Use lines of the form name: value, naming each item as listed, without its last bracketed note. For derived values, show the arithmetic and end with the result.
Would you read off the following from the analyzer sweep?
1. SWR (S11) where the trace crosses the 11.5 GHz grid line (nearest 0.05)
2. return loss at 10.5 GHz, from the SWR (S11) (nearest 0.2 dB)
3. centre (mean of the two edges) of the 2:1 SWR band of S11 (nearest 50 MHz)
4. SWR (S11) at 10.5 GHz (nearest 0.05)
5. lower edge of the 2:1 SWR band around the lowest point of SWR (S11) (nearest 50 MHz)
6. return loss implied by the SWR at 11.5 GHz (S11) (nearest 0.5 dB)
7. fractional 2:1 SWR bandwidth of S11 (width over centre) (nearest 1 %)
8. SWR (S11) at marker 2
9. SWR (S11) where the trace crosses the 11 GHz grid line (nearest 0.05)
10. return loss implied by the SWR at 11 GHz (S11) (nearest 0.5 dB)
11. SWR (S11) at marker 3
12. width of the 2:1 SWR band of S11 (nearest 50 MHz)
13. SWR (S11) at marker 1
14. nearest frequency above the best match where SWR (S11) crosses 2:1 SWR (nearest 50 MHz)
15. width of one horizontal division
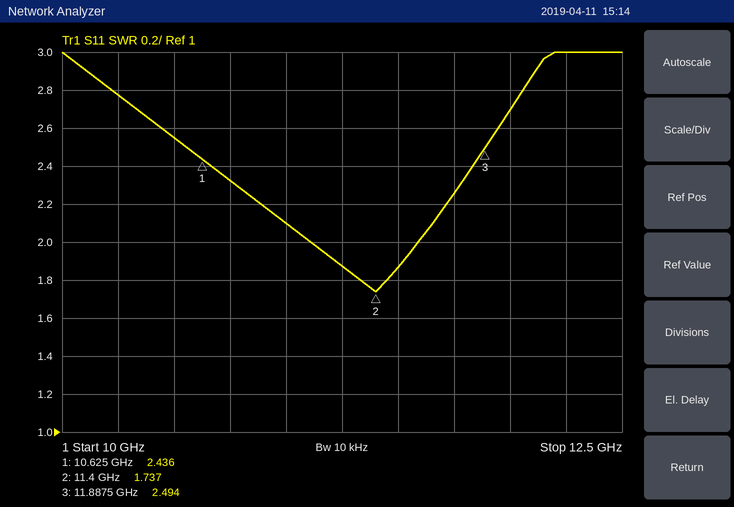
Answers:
SWR (S11) where the trace crosses the 11.5 GHz grid line: 1.85
return loss at 10.5 GHz, from the SWR (S11): −20 log10((2.55 − 1)/(2.55 + 1)) ≈ 7.2 dB
centre (mean of the two edges) of the 2:1 SWR band of S11: 11.35 GHz
SWR (S11) at 10.5 GHz: 2.55
lower edge of the 2:1 SWR band around the lowest point of SWR (S11): 11.10 GHz
return loss implied by the SWR at 11.5 GHz (S11): −20 log10((1.85 − 1)/(1.85 + 1)) ≈ 10.5 dB
fractional 2:1 SWR bandwidth of S11 (width over centre): 500 MHz / 11.35 GHz ≈ 4 %
SWR (S11) at marker 2: 1.737
SWR (S11) where the trace crosses the 11 GHz grid line: 2.10
return loss implied by the SWR at 11 GHz (S11): −20 log10((2.1 − 1)/(2.1 + 1)) ≈ 9.0 dB
SWR (S11) at marker 3: 2.494
width of the 2:1 SWR band of S11: 11.60 GHz − 11.10 GHz = 500 MHz
SWR (S11) at marker 1: 2.436
nearest frequency above the best match where SWR (S11) crosses 2:1 SWR: 11.60 GHz
width of one horizontal division: 250 MHz
